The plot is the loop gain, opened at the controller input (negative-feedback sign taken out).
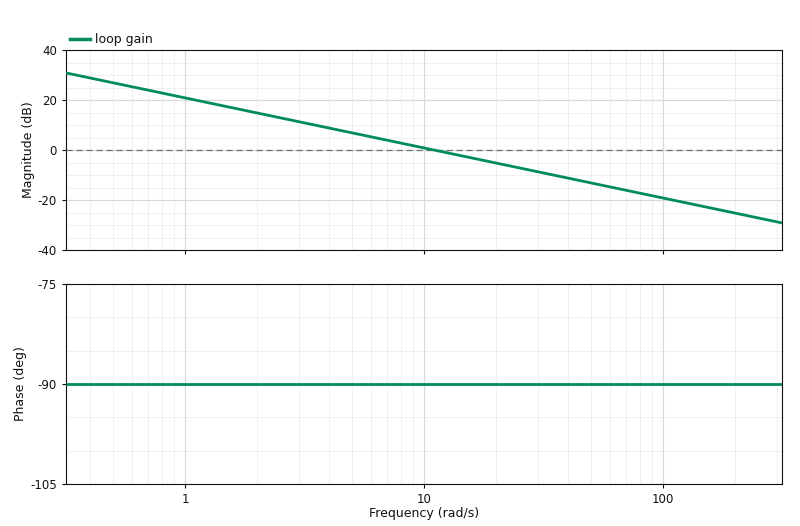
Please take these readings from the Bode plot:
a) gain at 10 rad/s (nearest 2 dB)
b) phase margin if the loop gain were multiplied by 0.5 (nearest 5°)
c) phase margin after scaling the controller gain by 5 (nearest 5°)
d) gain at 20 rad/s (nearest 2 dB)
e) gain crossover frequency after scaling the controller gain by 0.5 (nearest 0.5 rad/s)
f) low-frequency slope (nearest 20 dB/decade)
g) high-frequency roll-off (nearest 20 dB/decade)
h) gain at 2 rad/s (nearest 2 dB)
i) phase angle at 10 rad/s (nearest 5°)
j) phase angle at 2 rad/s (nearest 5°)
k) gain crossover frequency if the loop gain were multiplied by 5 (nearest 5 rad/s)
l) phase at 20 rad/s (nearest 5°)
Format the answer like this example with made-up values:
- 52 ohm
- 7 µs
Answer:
- 0 dB
- 90°
- 90°
- -6 dB
- 5.5 rad/s
- -20 dB/decade
- -20 dB/decade
- 14 dB
- -90°
- -90°
- 55 rad/s
- -90°
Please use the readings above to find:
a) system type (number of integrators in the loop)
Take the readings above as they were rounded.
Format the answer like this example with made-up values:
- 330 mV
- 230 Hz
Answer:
- 1
